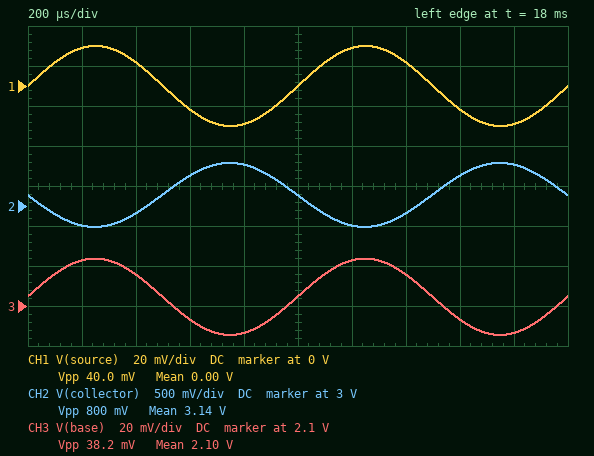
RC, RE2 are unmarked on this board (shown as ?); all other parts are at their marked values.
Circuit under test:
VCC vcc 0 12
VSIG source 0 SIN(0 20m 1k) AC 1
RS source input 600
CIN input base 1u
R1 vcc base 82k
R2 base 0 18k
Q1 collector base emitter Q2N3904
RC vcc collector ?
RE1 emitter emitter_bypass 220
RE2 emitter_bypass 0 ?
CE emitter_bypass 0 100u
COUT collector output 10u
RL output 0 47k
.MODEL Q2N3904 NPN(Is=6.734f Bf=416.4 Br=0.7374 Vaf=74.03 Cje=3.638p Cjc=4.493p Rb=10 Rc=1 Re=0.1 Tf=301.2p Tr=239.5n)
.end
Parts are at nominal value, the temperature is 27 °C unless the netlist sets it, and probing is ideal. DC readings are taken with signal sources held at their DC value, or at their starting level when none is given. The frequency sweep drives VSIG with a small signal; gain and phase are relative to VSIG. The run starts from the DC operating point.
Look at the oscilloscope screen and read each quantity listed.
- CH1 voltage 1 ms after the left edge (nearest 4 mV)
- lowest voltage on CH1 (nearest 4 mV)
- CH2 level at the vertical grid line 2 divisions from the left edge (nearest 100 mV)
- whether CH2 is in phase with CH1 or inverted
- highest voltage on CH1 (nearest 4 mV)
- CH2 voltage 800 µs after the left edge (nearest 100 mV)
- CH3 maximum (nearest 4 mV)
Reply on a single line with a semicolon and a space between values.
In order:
0 V; -20 mV; 2.9 V; inverted; 20 mV; 3.5 V; 2.124 V
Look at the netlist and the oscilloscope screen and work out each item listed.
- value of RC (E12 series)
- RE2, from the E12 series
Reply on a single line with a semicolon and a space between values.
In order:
5.6 kΩ; 680 Ω
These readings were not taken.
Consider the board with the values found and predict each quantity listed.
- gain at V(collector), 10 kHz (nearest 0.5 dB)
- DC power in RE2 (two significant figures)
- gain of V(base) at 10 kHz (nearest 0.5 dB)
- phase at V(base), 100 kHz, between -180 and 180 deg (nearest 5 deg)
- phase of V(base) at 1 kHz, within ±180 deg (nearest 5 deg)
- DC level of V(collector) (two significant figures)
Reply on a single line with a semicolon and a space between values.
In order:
26.0 dB; 1.7 mW; -0.5 dB; 0 deg; 0 deg; 3.1 V
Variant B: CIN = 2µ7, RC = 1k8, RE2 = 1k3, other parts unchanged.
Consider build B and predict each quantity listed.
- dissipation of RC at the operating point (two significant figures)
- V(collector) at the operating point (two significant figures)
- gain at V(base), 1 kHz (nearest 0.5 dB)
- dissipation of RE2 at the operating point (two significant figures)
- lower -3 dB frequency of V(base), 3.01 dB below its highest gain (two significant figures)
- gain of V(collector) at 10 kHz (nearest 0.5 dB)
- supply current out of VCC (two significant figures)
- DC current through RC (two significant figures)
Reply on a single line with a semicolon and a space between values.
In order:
1.7 mW; 10 V; -0.5 dB; 1.2 mW; 4.2 Hz; 16.5 dB; 1.1 mA; 960 µA
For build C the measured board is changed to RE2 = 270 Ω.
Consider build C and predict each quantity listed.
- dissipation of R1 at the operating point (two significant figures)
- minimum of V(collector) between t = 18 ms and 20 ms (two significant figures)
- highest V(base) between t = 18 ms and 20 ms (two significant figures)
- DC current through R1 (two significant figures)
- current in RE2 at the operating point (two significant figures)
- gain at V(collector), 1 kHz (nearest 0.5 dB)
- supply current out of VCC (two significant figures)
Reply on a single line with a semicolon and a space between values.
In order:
1.3 mW; 1.1 V; 1.7 V; 130 µA; 2.0 mA; -3.5 dB; 2.1 mA
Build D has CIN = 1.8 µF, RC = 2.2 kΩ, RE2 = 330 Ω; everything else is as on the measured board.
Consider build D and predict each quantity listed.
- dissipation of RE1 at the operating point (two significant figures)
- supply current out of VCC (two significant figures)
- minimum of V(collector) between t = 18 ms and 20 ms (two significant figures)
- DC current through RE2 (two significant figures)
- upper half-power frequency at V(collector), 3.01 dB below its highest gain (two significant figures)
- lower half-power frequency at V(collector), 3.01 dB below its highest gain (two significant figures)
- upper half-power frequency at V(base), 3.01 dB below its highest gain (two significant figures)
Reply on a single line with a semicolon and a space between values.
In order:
1.4 mW; 2.6 mA; 6.3 V; 2.5 mA; 8.0 MHz; 13 Hz; 8.6 MHz
